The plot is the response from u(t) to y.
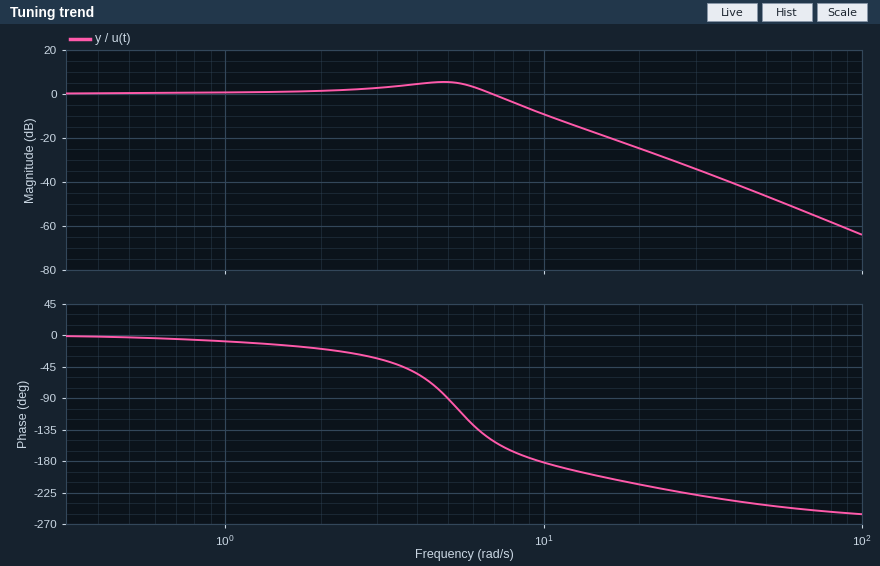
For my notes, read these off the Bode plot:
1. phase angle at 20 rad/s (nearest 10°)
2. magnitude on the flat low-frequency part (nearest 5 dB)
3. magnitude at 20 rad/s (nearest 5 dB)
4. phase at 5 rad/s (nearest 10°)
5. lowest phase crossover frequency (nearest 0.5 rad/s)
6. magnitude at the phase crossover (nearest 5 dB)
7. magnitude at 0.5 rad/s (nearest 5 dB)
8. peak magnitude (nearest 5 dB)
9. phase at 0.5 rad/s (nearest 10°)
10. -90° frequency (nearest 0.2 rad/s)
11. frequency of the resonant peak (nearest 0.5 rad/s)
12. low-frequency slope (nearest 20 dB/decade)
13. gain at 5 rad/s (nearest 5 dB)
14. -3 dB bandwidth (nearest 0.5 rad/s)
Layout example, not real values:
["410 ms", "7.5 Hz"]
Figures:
["-210°", "0 dB", "-25 dB", "-90°", "9.5 rad/s", "-10 dB", "0 dB", "5 dB", "0°", "5.0 rad/s", "5.0 rad/s", "0 dB/decade", "5 dB", "7.5 rad/s"]
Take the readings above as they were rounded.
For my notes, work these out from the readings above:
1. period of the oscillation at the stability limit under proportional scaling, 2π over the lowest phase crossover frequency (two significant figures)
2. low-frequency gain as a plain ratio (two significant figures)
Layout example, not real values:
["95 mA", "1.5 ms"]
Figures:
["0.66 s", "1.0"]
